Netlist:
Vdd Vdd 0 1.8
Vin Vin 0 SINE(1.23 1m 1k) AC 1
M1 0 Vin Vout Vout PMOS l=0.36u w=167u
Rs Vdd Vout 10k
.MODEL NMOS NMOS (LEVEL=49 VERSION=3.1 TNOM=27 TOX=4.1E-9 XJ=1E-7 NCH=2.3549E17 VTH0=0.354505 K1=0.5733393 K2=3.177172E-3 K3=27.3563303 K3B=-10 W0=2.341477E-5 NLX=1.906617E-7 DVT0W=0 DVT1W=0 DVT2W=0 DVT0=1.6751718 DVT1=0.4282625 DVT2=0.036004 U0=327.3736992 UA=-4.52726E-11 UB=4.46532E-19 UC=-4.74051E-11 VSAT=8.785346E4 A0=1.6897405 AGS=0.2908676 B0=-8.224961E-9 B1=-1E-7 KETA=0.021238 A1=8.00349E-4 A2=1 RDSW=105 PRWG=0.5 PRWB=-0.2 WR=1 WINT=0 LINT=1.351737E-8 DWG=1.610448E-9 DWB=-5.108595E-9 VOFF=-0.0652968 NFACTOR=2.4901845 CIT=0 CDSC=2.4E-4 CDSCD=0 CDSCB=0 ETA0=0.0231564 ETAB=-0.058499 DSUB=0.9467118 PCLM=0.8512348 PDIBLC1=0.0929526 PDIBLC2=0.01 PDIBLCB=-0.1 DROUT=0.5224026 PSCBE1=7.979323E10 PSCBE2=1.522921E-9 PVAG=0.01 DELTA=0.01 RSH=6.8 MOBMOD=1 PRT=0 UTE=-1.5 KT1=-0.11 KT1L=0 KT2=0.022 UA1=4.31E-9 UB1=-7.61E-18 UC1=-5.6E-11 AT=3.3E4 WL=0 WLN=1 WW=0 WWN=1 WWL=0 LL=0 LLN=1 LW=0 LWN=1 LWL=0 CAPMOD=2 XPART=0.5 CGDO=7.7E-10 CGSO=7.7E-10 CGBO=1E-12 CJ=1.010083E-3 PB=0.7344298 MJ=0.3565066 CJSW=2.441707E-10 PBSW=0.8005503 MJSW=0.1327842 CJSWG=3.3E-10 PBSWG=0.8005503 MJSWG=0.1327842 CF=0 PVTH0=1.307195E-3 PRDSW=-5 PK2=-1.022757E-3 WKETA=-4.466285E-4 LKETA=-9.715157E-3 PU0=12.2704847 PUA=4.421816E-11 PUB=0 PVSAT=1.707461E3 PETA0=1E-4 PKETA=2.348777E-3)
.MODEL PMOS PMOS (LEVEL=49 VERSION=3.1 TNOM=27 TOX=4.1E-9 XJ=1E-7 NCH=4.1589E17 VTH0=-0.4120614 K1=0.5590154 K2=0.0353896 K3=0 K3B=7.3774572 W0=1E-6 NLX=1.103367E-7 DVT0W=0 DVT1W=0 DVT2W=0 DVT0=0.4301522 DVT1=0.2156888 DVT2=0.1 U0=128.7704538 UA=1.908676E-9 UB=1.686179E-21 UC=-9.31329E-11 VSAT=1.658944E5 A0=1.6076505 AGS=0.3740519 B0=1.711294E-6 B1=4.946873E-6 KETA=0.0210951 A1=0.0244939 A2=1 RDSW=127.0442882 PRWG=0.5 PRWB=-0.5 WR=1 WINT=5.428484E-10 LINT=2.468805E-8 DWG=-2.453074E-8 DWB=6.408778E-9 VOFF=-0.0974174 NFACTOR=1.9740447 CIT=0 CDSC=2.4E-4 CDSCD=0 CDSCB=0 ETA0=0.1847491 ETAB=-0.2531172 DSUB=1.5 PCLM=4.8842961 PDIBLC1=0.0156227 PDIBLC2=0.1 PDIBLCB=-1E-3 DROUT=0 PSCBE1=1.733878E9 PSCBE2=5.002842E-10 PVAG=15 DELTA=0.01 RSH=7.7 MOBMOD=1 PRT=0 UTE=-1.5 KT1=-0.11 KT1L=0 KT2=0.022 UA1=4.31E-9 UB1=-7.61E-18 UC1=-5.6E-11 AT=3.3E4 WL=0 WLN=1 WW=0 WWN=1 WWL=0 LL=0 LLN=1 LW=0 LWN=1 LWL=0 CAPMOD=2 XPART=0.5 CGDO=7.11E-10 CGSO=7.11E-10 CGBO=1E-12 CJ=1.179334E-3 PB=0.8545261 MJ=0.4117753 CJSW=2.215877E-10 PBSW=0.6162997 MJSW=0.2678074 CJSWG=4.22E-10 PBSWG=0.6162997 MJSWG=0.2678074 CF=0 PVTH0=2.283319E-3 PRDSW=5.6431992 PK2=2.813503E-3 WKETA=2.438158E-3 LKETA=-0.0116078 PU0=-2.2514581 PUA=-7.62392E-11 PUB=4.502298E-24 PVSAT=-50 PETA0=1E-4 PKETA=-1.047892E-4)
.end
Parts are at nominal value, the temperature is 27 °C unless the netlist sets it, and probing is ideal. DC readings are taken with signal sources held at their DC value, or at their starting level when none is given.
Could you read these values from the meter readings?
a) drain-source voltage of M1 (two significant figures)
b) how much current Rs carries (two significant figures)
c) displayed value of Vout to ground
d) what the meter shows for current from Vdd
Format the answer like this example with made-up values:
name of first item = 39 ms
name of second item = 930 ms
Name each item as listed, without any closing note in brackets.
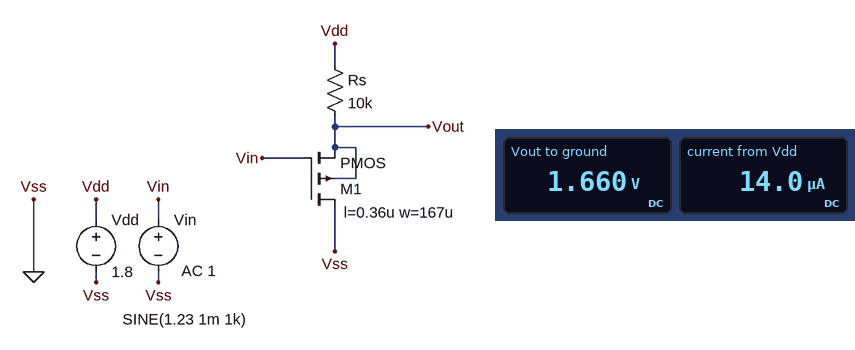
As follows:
drain-source voltage of M1 = -1.7 V
how much current Rs carries = 14 µA
displayed value of Vout to ground = 1.660 V
what the meter shows for current from Vdd = 14.0 µA
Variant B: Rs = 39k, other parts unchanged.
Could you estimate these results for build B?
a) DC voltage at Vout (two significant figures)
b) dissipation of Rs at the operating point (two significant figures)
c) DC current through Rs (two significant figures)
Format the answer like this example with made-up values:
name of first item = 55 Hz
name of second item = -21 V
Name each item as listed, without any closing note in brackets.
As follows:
DC voltage at Vout = 1.6 V
dissipation of Rs at the operating point = 900 nW
DC current through Rs = 4.8 µA
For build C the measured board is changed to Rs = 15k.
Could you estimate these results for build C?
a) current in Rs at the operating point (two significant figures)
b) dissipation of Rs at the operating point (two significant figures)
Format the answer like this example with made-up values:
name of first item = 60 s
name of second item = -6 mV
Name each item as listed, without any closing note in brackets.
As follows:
current in Rs at the operating point = 10 µA
dissipation of Rs at the operating point = 1.6 µW
